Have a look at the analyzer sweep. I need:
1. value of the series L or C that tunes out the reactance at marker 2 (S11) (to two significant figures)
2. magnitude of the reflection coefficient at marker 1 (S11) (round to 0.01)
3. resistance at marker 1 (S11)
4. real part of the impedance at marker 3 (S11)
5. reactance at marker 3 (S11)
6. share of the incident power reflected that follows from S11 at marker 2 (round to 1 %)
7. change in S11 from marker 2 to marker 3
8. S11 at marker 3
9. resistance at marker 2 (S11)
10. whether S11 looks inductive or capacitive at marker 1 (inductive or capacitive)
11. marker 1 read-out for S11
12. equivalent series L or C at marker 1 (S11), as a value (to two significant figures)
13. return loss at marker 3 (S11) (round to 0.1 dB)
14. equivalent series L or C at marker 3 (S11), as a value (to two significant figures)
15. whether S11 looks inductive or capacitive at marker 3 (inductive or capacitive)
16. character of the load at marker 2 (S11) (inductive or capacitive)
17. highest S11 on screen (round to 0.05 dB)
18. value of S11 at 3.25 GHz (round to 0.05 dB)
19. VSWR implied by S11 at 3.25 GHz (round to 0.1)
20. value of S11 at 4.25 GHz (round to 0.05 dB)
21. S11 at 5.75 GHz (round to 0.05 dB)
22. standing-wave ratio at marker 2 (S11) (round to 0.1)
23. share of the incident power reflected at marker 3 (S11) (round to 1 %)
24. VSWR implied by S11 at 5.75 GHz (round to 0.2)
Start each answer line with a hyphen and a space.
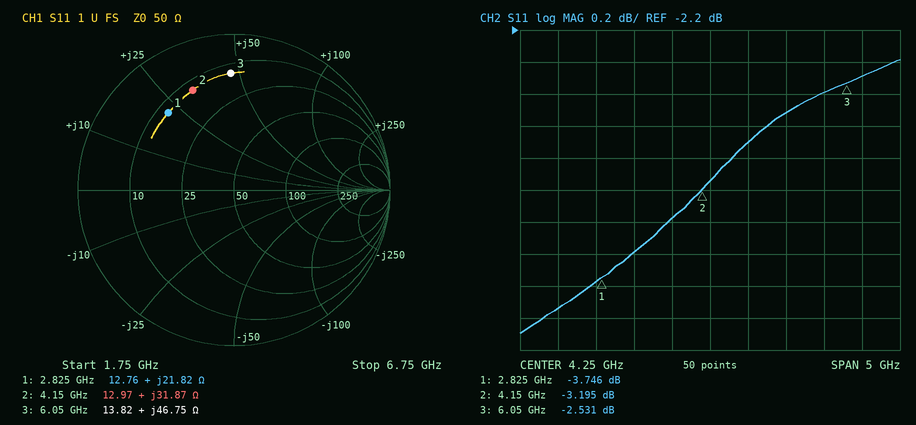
- 1.2 pF
- 0.65
- 12.76 Ω
- 13.82 Ω
- +46.75 Ω
- 48 %
- 0.664 dB
- -2.531 dB
- 12.97 Ω
- inductive
- -3.746 dB
- 1.2 nH
- 2.5 dB
- 1.2 nH
- inductive
- inductive
- -2.40 dB
- -3.60 dB
- 4.9
- -3.15 dB
- -2.60 dB
- 5.5
- 56 %
- 6.8
